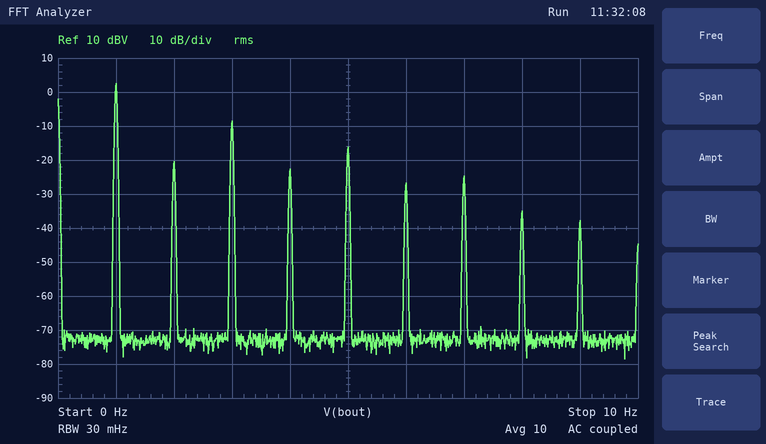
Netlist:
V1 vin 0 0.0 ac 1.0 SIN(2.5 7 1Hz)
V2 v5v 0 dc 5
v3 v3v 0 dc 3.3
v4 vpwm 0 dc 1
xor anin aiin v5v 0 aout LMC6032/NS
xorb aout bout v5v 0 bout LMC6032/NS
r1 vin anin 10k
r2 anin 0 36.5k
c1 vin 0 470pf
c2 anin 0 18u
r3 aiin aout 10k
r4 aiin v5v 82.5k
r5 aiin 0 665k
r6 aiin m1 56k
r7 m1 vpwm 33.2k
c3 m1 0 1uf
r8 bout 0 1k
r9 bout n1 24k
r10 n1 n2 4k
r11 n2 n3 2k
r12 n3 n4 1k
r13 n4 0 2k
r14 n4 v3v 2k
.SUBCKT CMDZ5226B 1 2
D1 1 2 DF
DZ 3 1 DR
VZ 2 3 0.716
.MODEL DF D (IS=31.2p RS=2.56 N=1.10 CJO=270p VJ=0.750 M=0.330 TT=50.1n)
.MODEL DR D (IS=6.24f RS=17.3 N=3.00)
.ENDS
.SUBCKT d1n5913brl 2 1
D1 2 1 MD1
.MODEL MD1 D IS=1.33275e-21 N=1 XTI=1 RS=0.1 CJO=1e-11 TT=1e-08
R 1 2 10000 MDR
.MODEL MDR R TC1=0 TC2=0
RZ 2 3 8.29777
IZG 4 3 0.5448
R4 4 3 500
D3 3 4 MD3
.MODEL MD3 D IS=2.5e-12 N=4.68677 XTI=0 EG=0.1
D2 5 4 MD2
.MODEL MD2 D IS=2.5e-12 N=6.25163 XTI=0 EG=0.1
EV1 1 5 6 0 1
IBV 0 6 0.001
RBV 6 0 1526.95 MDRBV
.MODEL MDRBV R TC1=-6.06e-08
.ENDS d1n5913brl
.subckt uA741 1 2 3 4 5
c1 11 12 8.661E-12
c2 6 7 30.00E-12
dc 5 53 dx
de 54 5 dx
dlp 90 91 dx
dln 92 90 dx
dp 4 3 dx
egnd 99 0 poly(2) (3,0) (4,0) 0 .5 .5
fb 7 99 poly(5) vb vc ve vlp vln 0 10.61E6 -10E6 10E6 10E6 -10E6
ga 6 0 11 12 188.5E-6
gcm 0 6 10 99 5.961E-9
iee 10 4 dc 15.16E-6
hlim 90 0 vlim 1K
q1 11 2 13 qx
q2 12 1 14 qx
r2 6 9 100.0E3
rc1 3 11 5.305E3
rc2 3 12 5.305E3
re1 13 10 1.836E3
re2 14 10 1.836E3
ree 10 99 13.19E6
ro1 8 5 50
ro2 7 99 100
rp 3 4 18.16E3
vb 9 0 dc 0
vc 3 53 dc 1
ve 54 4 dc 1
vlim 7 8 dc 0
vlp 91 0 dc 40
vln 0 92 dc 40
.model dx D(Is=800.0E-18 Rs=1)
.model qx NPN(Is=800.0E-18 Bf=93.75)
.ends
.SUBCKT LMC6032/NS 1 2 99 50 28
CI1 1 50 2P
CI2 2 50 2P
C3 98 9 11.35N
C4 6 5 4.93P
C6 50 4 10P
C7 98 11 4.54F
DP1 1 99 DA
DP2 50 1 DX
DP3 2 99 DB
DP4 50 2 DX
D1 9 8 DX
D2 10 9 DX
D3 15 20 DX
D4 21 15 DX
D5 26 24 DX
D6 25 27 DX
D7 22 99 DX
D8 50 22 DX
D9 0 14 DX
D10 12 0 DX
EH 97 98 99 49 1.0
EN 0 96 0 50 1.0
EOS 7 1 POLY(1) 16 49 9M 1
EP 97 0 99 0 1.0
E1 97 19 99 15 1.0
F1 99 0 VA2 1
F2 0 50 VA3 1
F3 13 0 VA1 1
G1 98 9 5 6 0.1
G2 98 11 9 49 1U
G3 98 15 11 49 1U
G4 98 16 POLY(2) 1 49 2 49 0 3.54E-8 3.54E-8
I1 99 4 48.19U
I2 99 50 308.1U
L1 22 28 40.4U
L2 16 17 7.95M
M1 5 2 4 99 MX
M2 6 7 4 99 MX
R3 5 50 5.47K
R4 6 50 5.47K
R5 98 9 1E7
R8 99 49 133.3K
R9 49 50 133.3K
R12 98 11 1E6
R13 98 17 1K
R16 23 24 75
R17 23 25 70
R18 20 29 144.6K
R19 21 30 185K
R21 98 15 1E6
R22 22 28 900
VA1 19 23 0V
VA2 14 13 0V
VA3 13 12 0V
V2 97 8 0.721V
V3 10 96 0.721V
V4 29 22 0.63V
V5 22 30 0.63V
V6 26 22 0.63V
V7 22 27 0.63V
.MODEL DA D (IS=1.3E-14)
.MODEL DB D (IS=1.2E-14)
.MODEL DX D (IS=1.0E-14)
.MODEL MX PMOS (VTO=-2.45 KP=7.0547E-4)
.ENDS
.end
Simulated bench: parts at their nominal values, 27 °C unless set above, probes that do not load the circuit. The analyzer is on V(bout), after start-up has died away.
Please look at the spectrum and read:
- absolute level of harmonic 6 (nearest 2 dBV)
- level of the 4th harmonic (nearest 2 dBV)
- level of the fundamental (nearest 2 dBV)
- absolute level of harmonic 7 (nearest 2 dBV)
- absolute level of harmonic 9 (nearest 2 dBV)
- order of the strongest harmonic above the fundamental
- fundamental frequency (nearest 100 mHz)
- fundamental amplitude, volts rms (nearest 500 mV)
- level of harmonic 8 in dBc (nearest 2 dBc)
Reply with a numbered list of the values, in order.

1. -26 dBV
2. -22 dBV
3. 2 dBV
4. -24 dBV
5. -38 dBV
6. 3
7. 1.0 Hz
8. 1.5 V
9. -38 dBc
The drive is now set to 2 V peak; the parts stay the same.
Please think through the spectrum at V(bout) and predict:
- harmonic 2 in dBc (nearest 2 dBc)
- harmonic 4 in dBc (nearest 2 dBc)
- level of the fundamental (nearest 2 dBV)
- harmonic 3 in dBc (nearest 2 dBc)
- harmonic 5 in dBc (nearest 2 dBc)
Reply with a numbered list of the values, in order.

1. -38 dBc
2. -40 dBc
3. 0 dBV
4. -40 dBc
5. -42 dBc
